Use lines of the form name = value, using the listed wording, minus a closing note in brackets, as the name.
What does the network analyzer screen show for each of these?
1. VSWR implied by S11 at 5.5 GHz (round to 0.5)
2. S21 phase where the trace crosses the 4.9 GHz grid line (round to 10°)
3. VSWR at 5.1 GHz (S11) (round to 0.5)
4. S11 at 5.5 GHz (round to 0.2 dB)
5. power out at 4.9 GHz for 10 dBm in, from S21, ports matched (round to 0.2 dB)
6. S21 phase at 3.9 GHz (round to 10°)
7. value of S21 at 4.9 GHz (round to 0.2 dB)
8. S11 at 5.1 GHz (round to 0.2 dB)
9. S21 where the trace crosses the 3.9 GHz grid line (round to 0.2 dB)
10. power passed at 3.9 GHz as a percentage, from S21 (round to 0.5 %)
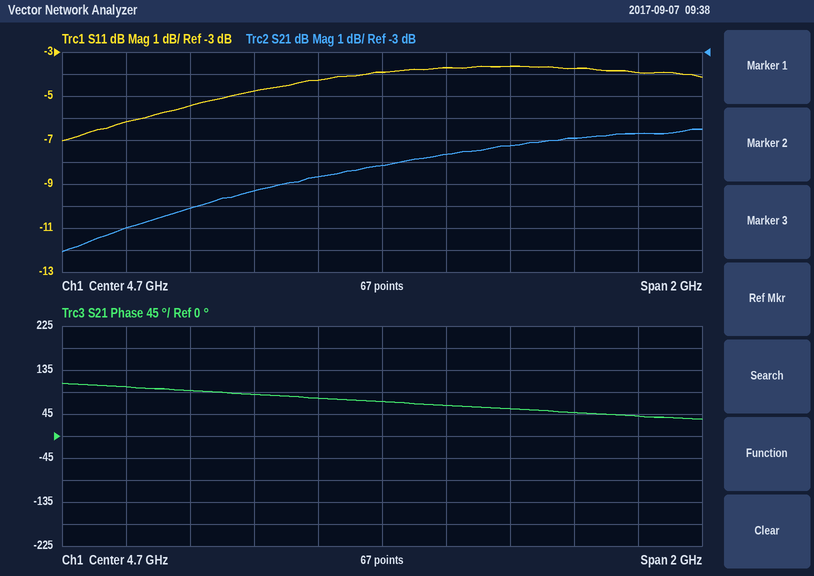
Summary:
VSWR implied by S11 at 5.5 GHz = 4.5
S21 phase where the trace crosses the 4.9 GHz grid line = 60°
VSWR at 5.1 GHz (S11) = 5.0
S11 at 5.5 GHz = -4.0 dB
power out at 4.9 GHz for 10 dBm in, from S21, ports matched = 2.4 dBm
S21 phase at 3.9 GHz = 100°
value of S21 at 4.9 GHz = -7.6 dB
S11 at 5.1 GHz = -3.6 dB
S21 where the trace crosses the 3.9 GHz grid line = -11.0 dB
power passed at 3.9 GHz as a percentage, from S21 = 8.0 %
